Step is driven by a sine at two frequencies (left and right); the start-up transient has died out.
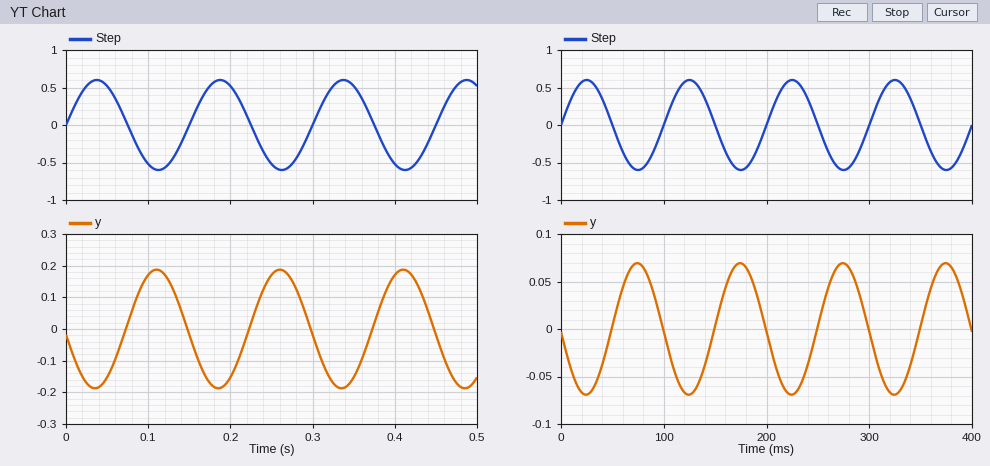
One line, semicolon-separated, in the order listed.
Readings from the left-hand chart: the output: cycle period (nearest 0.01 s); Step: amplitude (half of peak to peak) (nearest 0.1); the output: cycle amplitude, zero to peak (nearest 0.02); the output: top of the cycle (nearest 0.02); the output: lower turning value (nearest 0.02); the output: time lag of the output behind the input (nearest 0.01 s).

0.15 s; 0.6; 0.18; 0.18; -0.18; 0.07 s
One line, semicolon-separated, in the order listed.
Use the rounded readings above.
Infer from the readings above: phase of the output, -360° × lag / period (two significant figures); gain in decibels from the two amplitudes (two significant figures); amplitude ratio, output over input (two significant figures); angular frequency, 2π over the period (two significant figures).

-170°; -10 dB; 0.30; 42 rad/s
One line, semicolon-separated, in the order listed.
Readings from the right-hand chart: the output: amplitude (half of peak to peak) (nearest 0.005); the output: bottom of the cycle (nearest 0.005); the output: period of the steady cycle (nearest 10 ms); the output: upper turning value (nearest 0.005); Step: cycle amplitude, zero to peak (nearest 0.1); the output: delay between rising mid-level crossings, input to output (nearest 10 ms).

0.070; -0.070; 100 ms; 0.070; 0.6; 50 ms
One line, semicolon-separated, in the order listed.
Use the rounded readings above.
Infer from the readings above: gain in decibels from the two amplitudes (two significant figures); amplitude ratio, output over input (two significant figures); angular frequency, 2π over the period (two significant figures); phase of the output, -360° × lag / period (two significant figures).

-19 dB; 0.12; 0.063 rad/ms; -180°
